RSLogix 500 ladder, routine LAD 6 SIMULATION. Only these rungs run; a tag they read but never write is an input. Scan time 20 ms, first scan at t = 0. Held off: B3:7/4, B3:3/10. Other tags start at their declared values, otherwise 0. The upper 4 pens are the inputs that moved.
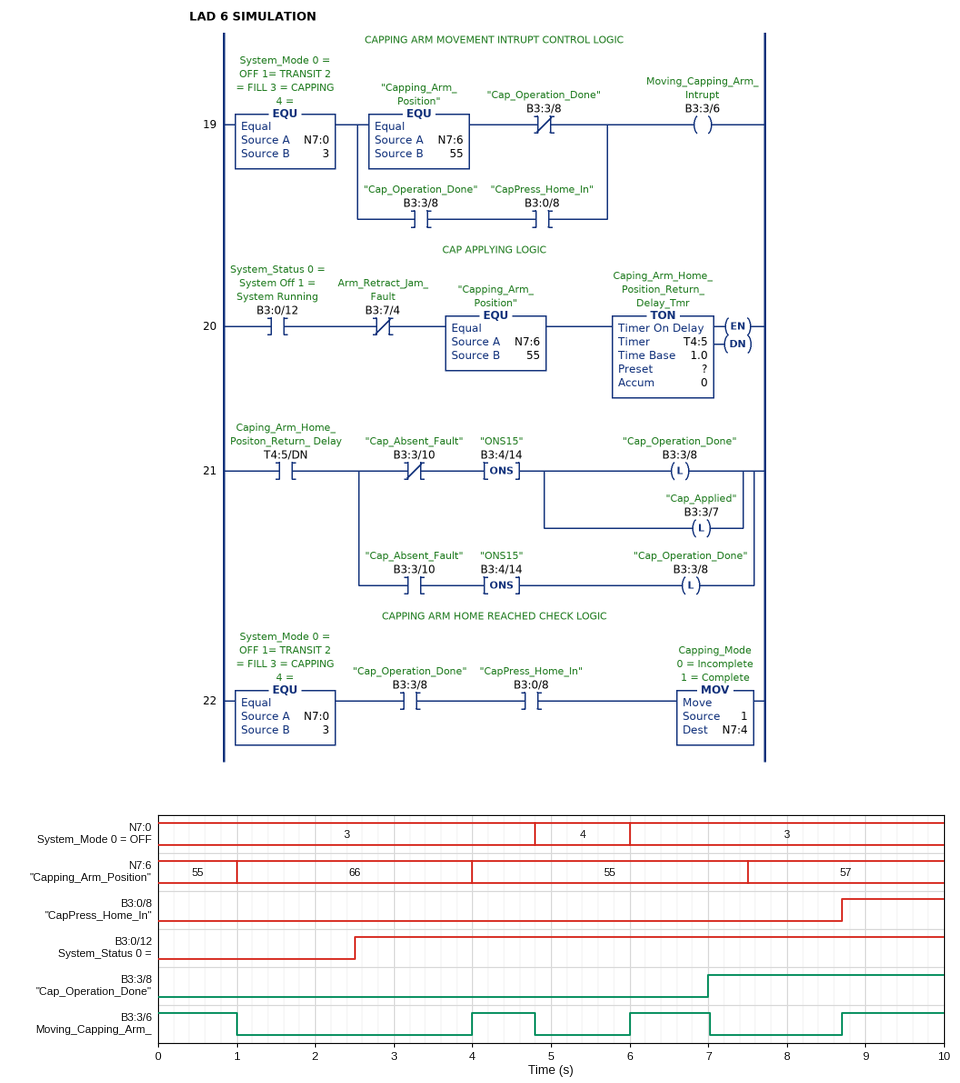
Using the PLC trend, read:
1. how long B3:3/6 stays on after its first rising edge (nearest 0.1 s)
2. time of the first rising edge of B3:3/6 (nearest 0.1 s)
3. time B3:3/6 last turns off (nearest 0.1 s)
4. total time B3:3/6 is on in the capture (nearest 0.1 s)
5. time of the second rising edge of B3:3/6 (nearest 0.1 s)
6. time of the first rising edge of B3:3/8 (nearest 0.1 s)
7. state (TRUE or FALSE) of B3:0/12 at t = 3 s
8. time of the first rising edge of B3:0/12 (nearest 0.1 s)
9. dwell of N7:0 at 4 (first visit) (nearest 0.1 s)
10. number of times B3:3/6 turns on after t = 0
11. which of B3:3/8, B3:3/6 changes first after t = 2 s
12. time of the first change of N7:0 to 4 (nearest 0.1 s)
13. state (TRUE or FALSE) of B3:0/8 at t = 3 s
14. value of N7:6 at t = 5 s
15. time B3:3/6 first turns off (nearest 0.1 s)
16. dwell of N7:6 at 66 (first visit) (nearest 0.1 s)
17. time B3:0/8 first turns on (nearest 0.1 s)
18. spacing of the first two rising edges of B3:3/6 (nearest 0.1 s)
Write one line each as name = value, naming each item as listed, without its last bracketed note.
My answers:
how long B3:3/6 stays on after its first rising edge = 0.8 s
time of the first rising edge of B3:3/6 = 4.0 s
time B3:3/6 last turns off = 7.0 s
total time B3:3/6 is on in the capture = 4.1 s
time of the second rising edge of B3:3/6 = 6.0 s
time of the first rising edge of B3:3/8 = 7.0 s
state (TRUE or FALSE) of B3:0/12 at t = 3 s = TRUE
time of the first rising edge of B3:0/12 = 2.5 s
dwell of N7:0 at 4 (first visit) = 1.2 s
number of times B3:3/6 turns on after t = 0 = 3
which of B3:3/8, B3:3/6 changes first after t = 2 s = B3:3/6
time of the first change of N7:0 to 4 = 4.8 s
state (TRUE or FALSE) of B3:0/8 at t = 3 s = FALSE
value of N7:6 at t = 5 s = 55
time B3:3/6 first turns off = 1.0 s
dwell of N7:6 at 66 (first visit) = 3.0 s
time B3:0/8 first turns on = 8.7 s
spacing of the first two rising edges of B3:3/6 = 2.0 s
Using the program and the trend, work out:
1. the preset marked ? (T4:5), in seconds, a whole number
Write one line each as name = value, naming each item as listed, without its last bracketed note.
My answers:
the preset marked ? (T4:5), in seconds, a whole number = 3 s
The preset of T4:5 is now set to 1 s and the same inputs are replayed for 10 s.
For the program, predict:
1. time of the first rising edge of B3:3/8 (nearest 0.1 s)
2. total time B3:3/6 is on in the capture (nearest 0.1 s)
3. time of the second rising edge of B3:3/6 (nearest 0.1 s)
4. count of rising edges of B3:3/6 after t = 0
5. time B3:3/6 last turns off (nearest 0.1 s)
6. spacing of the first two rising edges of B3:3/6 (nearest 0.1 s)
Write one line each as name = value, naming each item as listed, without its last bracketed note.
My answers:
time of the first rising edge of B3:3/8 = 5.0 s
total time B3:3/6 is on in the capture = 3.1 s
time of the second rising edge of B3:3/6 = 8.7 s
count of rising edges of B3:3/6 after t = 0 = 2
time B3:3/6 last turns off = 4.8 s
spacing of the first two rising edges of B3:3/6 = 4.7 s
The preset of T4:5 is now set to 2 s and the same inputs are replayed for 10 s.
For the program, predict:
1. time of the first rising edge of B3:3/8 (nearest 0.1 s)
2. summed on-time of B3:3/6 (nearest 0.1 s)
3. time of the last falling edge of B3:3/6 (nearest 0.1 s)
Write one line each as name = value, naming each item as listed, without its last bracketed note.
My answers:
time of the first rising edge of B3:3/8 = 6.0 s
summed on-time of B3:3/6 = 3.1 s
time of the last falling edge of B3:3/6 = 6.0 s
